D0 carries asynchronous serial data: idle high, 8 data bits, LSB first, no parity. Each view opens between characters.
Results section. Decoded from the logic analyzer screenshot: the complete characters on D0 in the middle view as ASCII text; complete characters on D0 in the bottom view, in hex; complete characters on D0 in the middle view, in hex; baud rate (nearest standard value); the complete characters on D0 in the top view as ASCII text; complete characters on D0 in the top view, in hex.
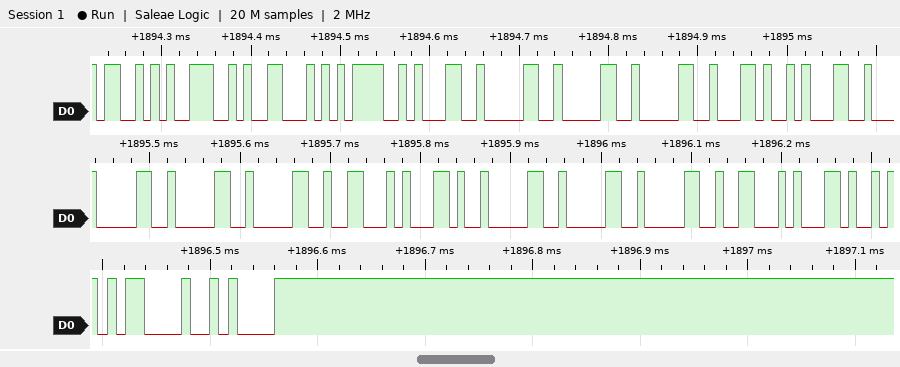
"000F,000F,"
0D, 0A
30, 30, 30, 46, 2C, 30, 30, 30, 46, 2C
115200 baud
"SNF=1000,1"
53, 4E, 46, 3D, 31, 30, 30, 30, 2C, 31
